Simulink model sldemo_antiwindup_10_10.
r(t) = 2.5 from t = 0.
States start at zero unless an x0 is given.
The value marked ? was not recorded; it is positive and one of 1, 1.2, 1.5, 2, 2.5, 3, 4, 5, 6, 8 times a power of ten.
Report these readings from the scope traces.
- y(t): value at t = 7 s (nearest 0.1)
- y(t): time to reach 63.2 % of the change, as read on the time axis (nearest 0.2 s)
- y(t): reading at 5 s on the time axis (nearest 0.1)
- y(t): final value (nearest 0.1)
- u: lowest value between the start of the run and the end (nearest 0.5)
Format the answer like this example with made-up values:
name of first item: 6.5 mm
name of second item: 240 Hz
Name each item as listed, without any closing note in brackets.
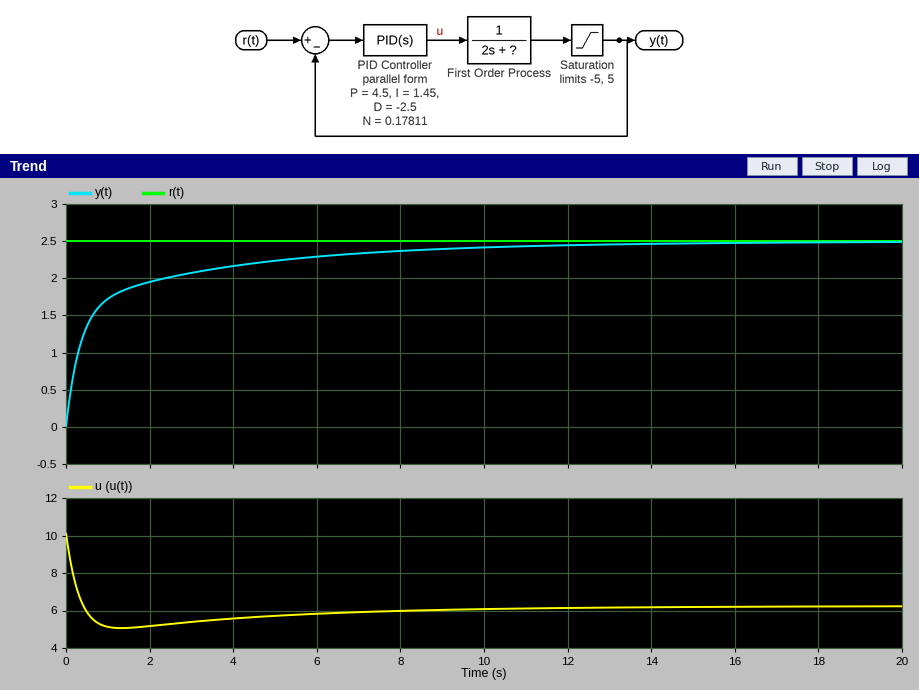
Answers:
y(t): value at t = 7 s: 2.3
y(t): time to reach 63.2 % of the change, as read on the time axis: 0.8 s
y(t): reading at 5 s on the time axis: 2.2
y(t): final value: 2.5
u: lowest value between the start of the run and the end: 5.0
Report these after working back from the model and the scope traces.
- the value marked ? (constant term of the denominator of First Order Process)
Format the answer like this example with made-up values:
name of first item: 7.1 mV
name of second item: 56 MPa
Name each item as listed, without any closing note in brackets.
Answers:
the value marked ?: 2.5
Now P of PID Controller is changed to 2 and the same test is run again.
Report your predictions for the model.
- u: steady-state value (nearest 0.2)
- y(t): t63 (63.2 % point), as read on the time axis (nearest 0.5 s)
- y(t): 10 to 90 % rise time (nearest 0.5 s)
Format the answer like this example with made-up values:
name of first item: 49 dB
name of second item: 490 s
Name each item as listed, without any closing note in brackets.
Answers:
u: steady-state value: 6.2
y(t): t63 (63.2 % point), as read on the time axis: 1.5 s
y(t): 10 to 90 % rise time: 4.0 s
